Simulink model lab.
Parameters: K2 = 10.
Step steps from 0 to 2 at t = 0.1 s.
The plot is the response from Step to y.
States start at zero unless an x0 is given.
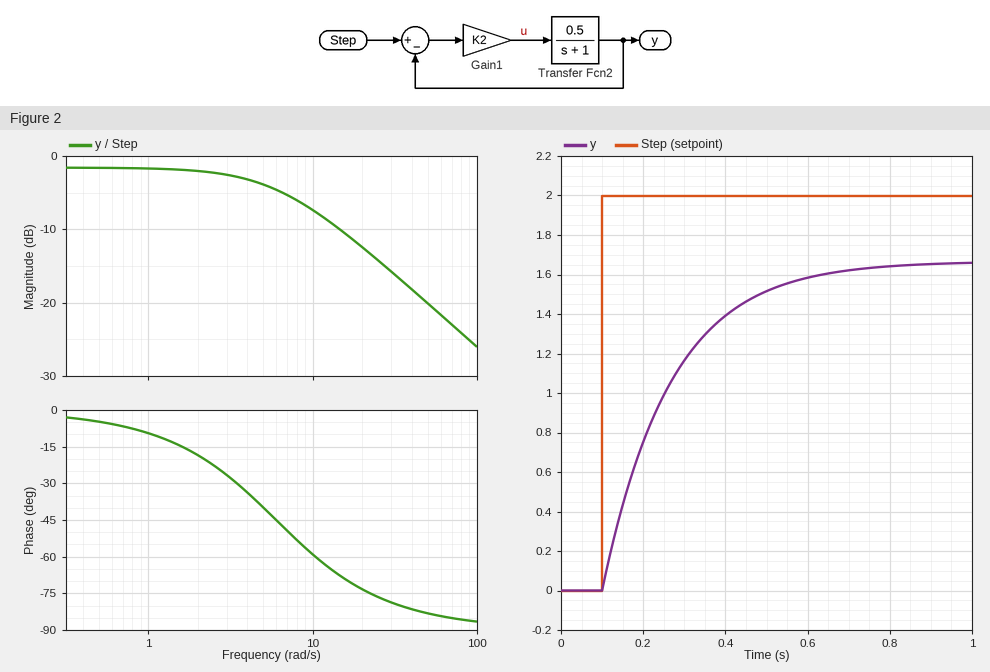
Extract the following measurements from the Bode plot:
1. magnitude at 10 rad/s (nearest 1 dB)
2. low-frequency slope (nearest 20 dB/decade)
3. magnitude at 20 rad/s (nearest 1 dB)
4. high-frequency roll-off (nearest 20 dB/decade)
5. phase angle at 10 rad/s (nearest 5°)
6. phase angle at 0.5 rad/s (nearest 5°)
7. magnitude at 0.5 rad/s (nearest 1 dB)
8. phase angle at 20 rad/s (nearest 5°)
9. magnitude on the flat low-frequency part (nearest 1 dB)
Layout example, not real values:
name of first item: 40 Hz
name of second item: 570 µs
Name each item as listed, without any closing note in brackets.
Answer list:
magnitude at 10 rad/s: -7 dB
low-frequency slope: 0 dB/decade
magnitude at 20 rad/s: -12 dB
high-frequency roll-off: -20 dB/decade
phase angle at 10 rad/s: -60°
phase angle at 0.5 rad/s: -5°
magnitude at 0.5 rad/s: -2 dB
phase angle at 20 rad/s: -75°
magnitude on the flat low-frequency part: -2 dB
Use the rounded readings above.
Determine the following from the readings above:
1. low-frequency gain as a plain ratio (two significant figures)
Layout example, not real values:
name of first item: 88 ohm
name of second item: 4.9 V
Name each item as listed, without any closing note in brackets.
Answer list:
low-frequency gain as a plain ratio: 0.79
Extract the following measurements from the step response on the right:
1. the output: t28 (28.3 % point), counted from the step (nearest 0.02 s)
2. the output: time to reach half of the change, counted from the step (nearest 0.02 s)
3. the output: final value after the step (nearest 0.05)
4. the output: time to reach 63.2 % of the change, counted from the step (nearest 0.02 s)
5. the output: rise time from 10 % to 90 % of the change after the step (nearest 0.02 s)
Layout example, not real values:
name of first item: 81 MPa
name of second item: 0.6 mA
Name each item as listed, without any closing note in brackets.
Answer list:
the output: t28 (28.3 % point), counted from the step: 0.06 s
the output: time to reach half of the change, counted from the step: 0.12 s
the output: final value after the step: 1.65
the output: time to reach 63.2 % of the change, counted from the step: 0.16 s
the output: rise time from 10 % to 90 % of the change after the step: 0.36 s
